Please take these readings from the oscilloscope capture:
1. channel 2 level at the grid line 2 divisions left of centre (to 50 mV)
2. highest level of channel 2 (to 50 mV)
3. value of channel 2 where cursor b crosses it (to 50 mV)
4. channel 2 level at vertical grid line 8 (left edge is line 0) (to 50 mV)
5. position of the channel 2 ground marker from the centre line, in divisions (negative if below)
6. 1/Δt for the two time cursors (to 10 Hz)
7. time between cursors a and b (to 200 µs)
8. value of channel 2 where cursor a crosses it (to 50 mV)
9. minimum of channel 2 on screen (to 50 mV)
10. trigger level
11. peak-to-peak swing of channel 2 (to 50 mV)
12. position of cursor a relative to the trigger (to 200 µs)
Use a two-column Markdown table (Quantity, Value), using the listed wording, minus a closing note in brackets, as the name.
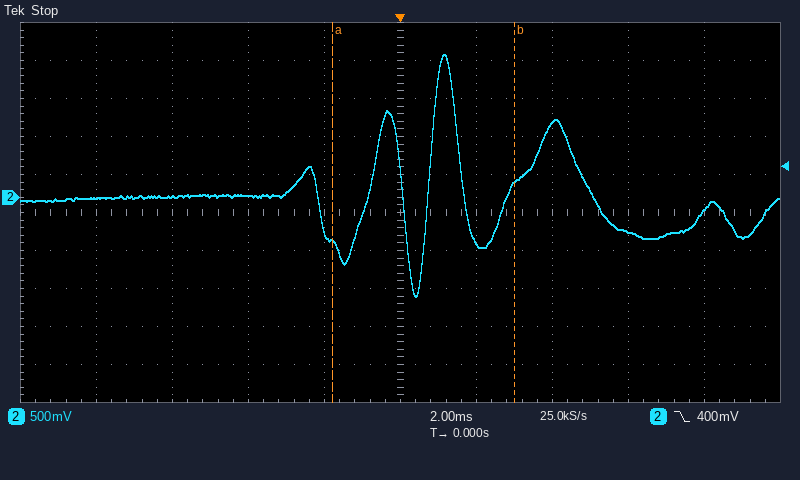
| Quantity | Value |
|---|---|
| channel 2 level at the grid line 2 divisions left of centre | 0 mV |
| highest level of channel 2 | 1.90 V |
| value of channel 2 where cursor b crosses it | 200 mV |
| channel 2 level at vertical grid line 8 (left edge is line 0) | -450 mV |
| position of the channel 2 ground marker from the centre line, in divisions | +0.4 div |
| 1/Δt for the two time cursors | 210 Hz |
| time between cursors a and b | 4.8 ms |
| value of channel 2 where cursor a crosses it | -600 mV |
| minimum of channel 2 on screen | -1.30 V |
| trigger level | 400 mV |
| peak-to-peak swing of channel 2 | 3.20 V |
| position of cursor a relative to the trigger | -1.8 ms |
